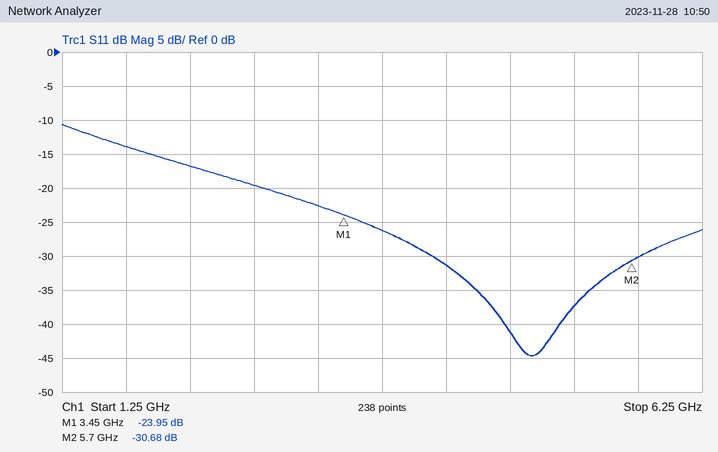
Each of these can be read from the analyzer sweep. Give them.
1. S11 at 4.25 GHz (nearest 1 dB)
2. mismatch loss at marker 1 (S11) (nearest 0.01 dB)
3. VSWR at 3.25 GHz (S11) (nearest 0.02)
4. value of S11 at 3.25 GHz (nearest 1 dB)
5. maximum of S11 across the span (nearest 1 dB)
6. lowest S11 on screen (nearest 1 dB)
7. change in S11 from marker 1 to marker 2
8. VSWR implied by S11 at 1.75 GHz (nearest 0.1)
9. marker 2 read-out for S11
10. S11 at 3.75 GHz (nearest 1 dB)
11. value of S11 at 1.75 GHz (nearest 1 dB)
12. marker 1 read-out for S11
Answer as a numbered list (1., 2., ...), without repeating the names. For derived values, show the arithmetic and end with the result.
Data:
1. -31 dB
2. −10 log10(1 − 10^(-23.95/10)) ≈ 0.02 dB
3. |Γ| = 10^(-23/20) = 0.0708; VSWR = (1 + 0.0708)/(1 − 0.0708) ≈ 1.15, so 1.16 to the nearest 0.02
4. -23 dB
5. -11 dB
6. -45 dB
7. -30.68 − (-23.95) = -6.73 dB
8. |Γ| = 10^(-14/20) = 0.1995; VSWR = (1 + 0.1995)/(1 − 0.1995) ≈ 1.5
9. -30.68 dB
10. -26 dB
11. -14 dB
12. -23.95 dB
